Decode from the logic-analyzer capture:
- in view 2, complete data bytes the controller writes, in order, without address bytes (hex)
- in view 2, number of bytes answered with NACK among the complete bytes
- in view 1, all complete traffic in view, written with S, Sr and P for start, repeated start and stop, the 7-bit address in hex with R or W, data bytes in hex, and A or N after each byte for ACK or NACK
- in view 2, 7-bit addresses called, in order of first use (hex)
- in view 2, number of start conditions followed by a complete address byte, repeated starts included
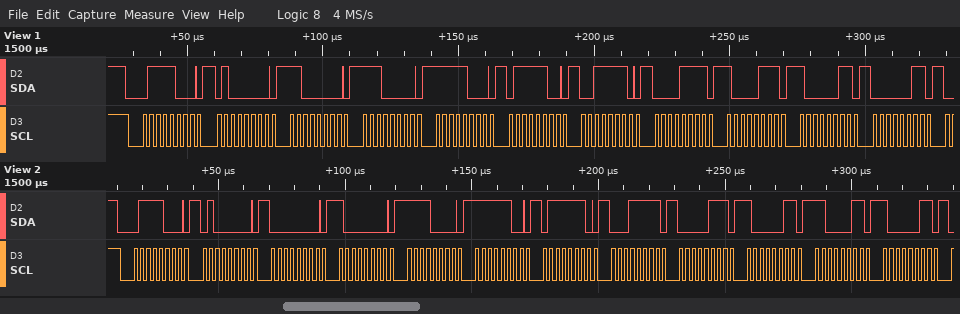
40 00 80 F0 FC 7E 1F 07 83 C3 83
0
S 3CW A 40 A C0 A E0 A F8 A 7C A 3E A 0F A 87 A 83 A 03 A
0x3C
1
